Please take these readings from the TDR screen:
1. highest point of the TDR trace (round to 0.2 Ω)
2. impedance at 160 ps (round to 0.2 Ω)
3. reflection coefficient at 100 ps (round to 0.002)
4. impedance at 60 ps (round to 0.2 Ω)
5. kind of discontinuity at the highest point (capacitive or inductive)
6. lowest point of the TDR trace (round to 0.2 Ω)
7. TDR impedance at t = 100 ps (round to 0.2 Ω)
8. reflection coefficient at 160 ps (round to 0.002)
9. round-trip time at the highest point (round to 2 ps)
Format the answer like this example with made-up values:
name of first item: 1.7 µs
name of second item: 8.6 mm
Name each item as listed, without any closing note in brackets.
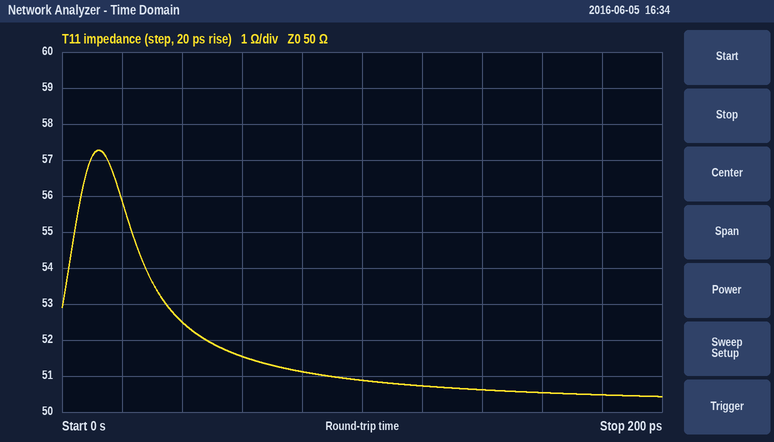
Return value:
highest point of the TDR trace: 57.2 Ω
impedance at 160 ps: 50.6 Ω
reflection coefficient at 100 ps: +0.008
impedance at 60 ps: 51.6 Ω
kind of discontinuity at the highest point: inductive
lowest point of the TDR trace: 50.4 Ω
TDR impedance at t = 100 ps: 50.8 Ω
reflection coefficient at 160 ps: +0.006
round-trip time at the highest point: 12 ps
